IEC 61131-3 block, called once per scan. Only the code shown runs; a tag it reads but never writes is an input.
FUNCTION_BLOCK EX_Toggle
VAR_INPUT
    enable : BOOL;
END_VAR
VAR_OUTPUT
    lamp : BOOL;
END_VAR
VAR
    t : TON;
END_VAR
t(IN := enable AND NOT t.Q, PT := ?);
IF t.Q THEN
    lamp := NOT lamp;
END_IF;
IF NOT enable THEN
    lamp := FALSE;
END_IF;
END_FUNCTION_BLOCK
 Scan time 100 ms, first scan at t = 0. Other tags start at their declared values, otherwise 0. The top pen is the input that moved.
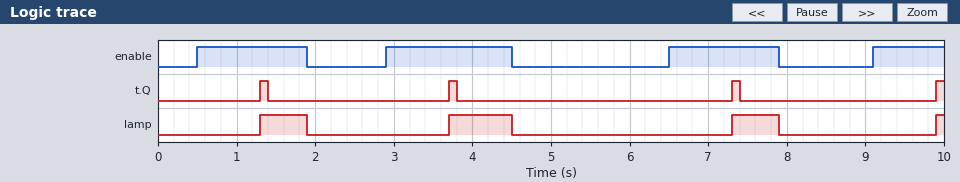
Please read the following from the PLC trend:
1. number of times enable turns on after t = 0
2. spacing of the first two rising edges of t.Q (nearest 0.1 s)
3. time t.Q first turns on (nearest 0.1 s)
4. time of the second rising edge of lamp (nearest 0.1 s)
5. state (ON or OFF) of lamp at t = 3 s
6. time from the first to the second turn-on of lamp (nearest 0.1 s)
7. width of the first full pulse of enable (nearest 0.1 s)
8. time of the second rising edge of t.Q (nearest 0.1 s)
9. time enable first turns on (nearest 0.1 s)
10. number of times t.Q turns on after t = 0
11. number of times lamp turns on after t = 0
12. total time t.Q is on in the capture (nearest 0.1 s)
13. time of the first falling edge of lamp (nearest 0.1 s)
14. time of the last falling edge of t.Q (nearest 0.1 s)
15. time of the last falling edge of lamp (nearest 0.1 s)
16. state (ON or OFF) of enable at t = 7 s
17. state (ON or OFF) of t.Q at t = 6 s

4
2.4 s
1.3 s
3.7 s
OFF
2.4 s
1.4 s
3.7 s
0.5 s
4
4
0.4 s
1.9 s
7.4 s
7.9 s
ON
OFF
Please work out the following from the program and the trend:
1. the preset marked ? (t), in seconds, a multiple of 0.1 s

0.8 s
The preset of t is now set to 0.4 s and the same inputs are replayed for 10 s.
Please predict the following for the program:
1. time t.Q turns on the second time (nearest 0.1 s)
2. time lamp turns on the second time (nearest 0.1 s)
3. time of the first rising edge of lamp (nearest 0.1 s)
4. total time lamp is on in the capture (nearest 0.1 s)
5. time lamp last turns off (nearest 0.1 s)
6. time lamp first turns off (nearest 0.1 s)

1.5 s
3.3 s
0.9 s
2.3 s
7.5 s
1.5 s
